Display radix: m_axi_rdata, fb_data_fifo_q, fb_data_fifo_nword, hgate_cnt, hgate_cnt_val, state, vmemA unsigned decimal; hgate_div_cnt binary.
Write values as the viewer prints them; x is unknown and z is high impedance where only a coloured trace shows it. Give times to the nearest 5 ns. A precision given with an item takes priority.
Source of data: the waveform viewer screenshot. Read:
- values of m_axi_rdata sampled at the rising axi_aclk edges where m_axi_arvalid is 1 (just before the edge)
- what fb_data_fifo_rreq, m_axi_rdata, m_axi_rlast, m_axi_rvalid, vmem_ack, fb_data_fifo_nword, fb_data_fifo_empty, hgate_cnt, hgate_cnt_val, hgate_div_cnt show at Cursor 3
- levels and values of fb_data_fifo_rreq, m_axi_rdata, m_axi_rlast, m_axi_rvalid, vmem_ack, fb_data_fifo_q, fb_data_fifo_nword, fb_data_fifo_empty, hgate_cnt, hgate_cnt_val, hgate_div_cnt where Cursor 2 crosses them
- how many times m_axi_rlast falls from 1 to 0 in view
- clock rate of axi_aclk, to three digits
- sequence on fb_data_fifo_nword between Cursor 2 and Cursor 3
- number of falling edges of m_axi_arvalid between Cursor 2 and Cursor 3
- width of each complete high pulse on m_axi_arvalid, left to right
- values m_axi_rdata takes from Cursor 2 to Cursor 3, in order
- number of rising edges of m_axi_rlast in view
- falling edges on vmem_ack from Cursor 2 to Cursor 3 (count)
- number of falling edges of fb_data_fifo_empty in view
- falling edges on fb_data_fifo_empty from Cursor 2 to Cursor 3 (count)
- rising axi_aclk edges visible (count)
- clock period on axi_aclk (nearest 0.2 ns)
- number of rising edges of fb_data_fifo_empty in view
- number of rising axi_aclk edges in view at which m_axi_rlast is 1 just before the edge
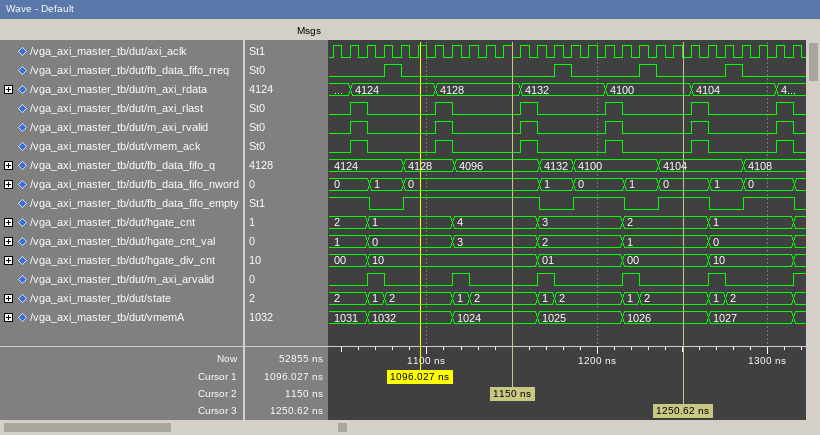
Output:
4124, 4128, 4132, 4100, 4104
fb_data_fifo_rreq=0, m_axi_rdata=4100, m_axi_rlast=0, m_axi_rvalid=0, vmem_ack=0, fb_data_fifo_nword=0, fb_data_fifo_empty=1, hgate_cnt=2, hgate_cnt_val=1, hgate_div_cnt=00
fb_data_fifo_rreq=0, m_axi_rdata=4128, m_axi_rlast=0, m_axi_rvalid=0, vmem_ack=0, fb_data_fifo_q=4096, fb_data_fifo_nword=0, fb_data_fifo_empty=1, hgate_cnt=4, hgate_cnt_val=3, hgate_div_cnt=10
6
100 MHz
0, 1, 0, 1, 0
2
10 ns, 10 ns, 10 ns, 10 ns, 10 ns
4128, 4132, 4100
6
2
5
2
28
10 ns
4
6
